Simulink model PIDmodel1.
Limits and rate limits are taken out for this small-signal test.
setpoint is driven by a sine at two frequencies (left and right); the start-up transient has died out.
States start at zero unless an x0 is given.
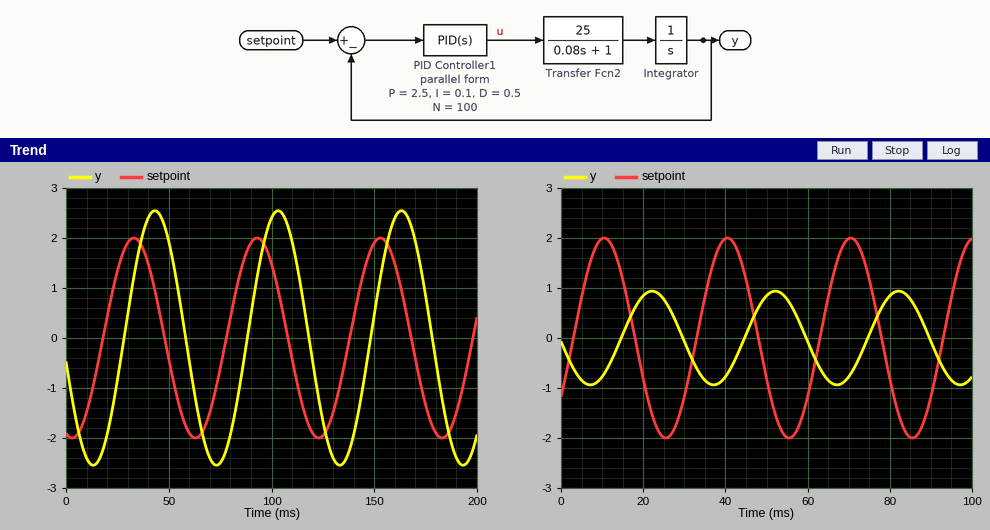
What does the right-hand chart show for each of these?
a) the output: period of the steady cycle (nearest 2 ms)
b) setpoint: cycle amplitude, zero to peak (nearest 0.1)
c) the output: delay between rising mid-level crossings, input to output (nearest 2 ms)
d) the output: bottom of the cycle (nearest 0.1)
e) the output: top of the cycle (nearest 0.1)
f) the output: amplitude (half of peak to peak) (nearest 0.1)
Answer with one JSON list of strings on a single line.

["30 ms", "2.0", "12 ms", "-0.9", "0.9", "0.9"]
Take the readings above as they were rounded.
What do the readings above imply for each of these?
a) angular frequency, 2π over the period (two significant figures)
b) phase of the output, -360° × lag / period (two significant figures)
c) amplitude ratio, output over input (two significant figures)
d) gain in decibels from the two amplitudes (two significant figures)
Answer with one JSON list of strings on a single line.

["0.21 rad/ms", "-140°", "0.45", "-6.9 dB"]
